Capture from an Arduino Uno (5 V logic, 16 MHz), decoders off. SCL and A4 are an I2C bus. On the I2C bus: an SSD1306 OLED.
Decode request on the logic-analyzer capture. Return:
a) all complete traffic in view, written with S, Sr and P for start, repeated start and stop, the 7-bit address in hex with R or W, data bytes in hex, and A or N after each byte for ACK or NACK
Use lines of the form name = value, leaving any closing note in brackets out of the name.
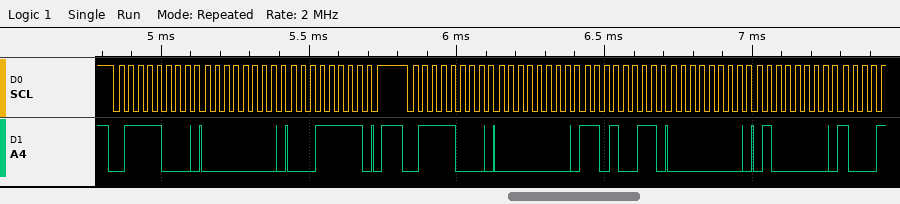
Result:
all complete traffic in view, written with S, Sr and P for start, repeated start and stop, the 7-bit address in hex with R or W, data bytes in hex, and A or N after each byte for ACK or NACK = S 3CW A 00 A 1F A P S 3CW A 00 A D3 A 00 A 40 A
